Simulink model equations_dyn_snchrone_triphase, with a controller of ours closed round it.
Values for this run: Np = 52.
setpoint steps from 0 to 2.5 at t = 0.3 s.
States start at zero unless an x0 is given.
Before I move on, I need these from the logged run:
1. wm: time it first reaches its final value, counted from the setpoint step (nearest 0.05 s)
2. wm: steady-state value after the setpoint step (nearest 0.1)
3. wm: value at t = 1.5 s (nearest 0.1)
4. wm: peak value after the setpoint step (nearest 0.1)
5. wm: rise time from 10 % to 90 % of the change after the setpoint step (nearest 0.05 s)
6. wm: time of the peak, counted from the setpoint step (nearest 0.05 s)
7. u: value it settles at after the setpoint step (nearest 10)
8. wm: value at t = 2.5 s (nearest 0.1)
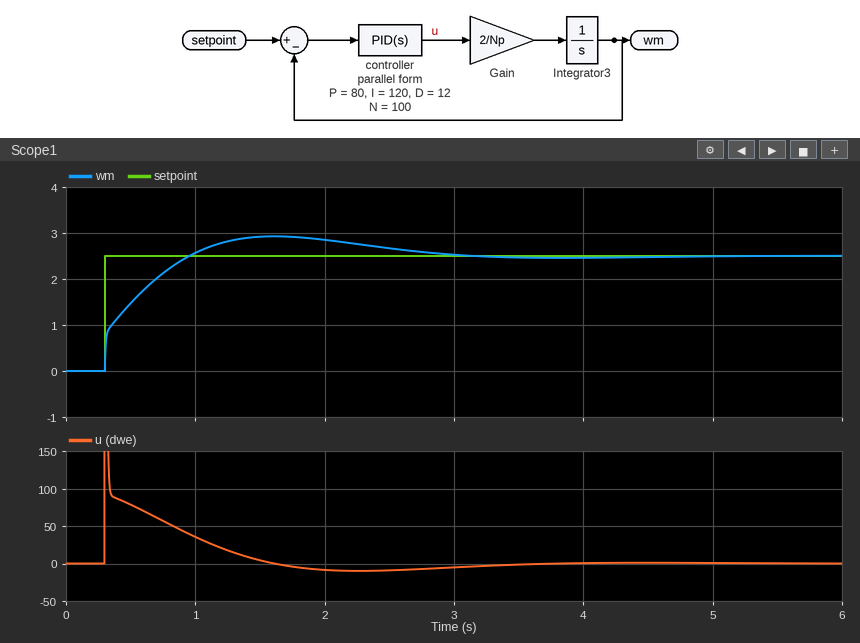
0.65 s
2.5
2.9
2.9
0.50 s
1.30 s
0
2.7
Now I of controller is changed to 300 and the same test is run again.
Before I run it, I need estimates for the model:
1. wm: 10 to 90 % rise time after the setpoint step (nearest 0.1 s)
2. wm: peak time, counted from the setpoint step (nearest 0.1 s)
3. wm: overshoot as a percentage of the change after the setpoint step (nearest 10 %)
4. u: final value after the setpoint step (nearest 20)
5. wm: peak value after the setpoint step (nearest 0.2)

0.4 s
0.9 s
30 %
0
3.2
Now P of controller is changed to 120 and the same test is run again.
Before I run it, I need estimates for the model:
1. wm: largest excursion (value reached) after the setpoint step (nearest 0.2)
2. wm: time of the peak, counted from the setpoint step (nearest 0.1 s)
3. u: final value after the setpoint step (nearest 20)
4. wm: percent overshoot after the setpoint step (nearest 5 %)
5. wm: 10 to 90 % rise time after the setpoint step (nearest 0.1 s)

2.8
1.2 s
0
10 %
0.4 s
